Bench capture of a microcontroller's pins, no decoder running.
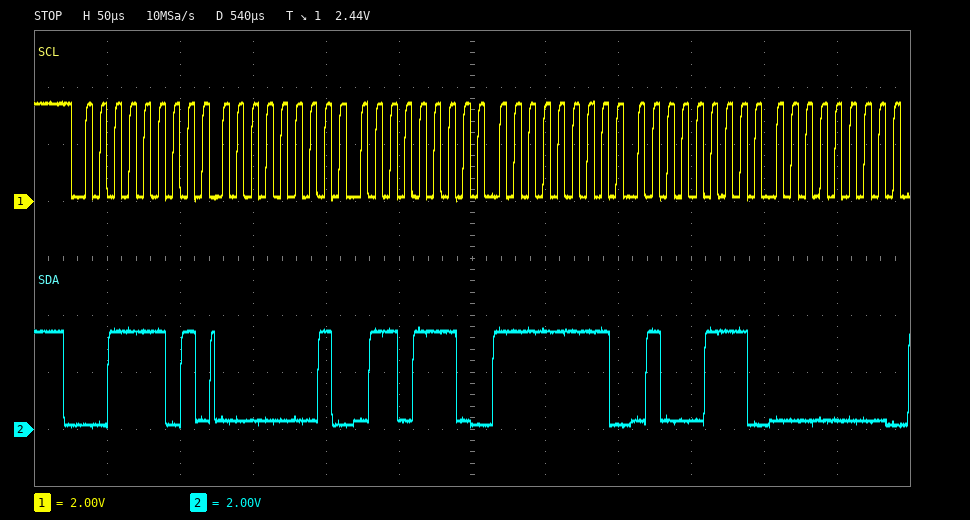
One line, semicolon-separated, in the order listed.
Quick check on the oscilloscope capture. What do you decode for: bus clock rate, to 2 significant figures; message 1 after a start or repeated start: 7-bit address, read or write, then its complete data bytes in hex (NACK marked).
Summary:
100 kHz; 0x1E read: 01 6E FF 47 00
